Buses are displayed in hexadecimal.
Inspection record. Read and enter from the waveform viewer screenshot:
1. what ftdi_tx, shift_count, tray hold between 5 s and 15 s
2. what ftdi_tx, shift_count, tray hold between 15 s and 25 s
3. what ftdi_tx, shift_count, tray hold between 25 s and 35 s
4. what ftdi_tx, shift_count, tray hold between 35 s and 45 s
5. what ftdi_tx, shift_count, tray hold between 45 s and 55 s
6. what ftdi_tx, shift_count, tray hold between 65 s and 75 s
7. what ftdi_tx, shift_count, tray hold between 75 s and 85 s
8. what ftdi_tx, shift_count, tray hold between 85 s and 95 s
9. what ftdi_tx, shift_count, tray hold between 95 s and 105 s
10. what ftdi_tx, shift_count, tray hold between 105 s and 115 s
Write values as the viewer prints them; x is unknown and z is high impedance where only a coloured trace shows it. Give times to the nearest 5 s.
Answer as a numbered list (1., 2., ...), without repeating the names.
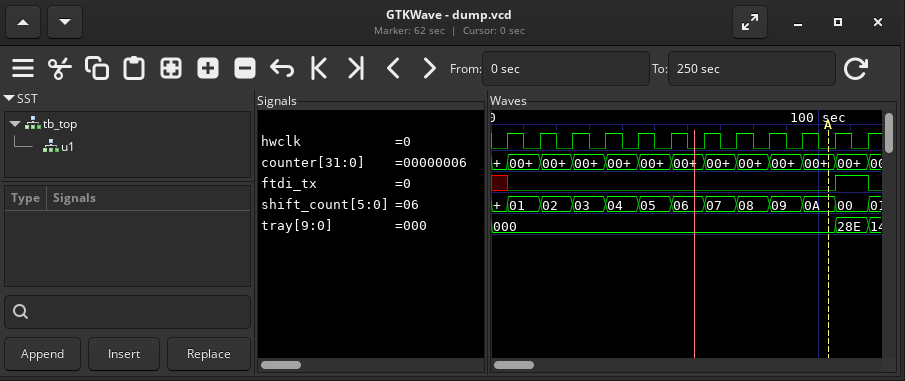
1. ftdi_tx=0, shift_count=01, tray=000
2. ftdi_tx=0, shift_count=02, tray=000
3. ftdi_tx=0, shift_count=03, tray=000
4. ftdi_tx=0, shift_count=04, tray=000
5. ftdi_tx=0, shift_count=05, tray=000
6. ftdi_tx=0, shift_count=07, tray=000
7. ftdi_tx=0, shift_count=08, tray=000
8. ftdi_tx=0, shift_count=09, tray=000
9. ftdi_tx=0, shift_count=0A, tray=000
10. ftdi_tx=1, shift_count=00, tray=28E
